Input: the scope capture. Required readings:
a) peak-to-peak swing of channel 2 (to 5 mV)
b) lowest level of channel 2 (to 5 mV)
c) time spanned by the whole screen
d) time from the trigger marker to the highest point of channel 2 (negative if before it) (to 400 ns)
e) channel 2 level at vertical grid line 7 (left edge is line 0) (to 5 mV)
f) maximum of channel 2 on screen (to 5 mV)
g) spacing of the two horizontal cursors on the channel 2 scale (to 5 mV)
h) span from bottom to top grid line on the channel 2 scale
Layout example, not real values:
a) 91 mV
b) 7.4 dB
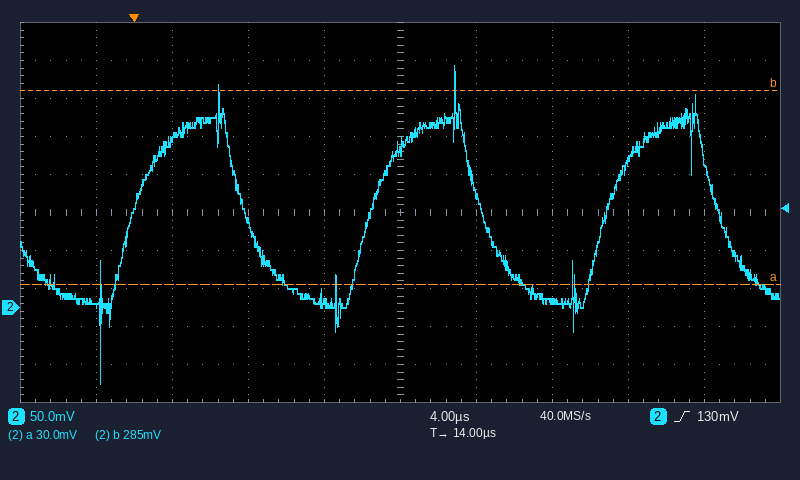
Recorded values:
a) 420 mV
b) -100 mV
c) 40 µs
d) +16.8 µs
e) 10 mV
f) 320 mV
g) 255 mV
h) 500 mV
